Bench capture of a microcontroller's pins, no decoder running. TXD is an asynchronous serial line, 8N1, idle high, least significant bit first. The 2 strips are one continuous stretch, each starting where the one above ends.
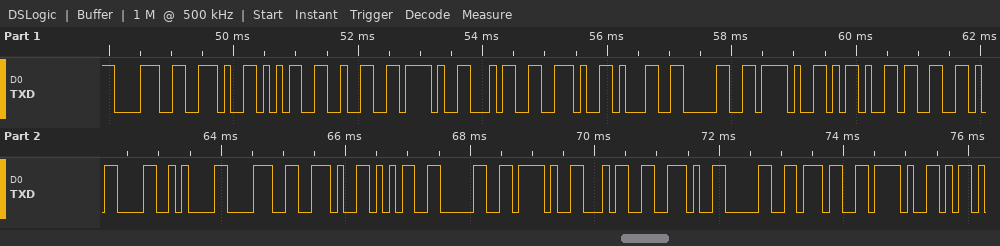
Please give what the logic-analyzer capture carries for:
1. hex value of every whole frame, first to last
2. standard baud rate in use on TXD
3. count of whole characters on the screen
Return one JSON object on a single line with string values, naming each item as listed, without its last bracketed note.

{"hex value of every whole frame, first to last": "38 2E 35 32 2F 34 2E 31 30 2F 2D 33 0D 0A 38 2E 35 30 2F 34 2E 30 37 2F", "standard baud rate in use on TXD": "9600 baud", "count of whole characters on the screen": "24"}
